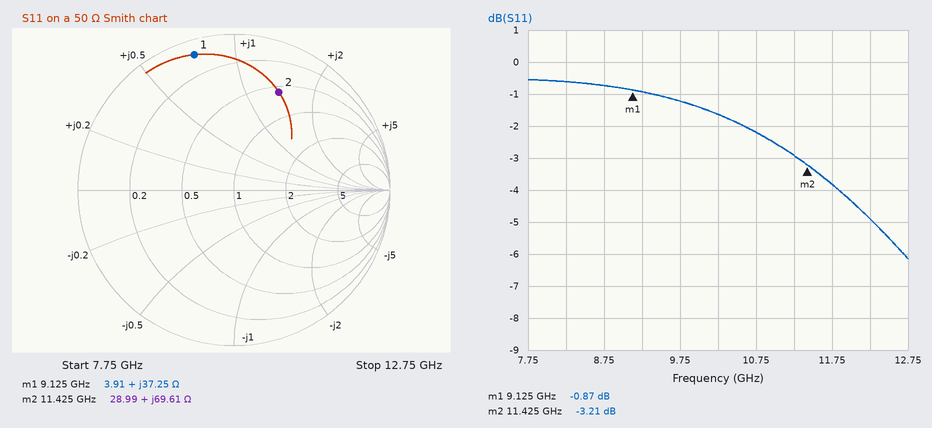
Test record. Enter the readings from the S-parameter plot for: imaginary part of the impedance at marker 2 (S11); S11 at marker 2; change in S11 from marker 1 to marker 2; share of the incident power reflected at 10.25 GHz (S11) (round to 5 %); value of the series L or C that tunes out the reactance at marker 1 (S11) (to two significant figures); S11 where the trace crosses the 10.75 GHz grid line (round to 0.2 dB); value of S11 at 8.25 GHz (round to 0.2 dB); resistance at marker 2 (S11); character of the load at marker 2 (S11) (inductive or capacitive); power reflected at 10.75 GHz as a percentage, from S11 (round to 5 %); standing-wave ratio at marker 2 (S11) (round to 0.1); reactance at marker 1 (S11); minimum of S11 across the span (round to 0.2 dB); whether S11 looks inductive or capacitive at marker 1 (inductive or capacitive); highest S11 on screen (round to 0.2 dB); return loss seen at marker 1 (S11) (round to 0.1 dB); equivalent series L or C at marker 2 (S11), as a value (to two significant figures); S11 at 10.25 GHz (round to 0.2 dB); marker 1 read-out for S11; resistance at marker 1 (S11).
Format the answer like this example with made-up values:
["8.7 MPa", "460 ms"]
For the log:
["+69.61 Ω", "-3.21 dB", "-2.34 dB", "70 %", "470 fF", "-2.2 dB", "-0.6 dB", "28.99 Ω", "inductive", "60 %", "5.5", "+37.25 Ω", "-6.2 dB", "inductive", "-0.6 dB", "0.9 dB", "970 pH", "-1.6 dB", "-0.87 dB", "3.91 Ω"]
